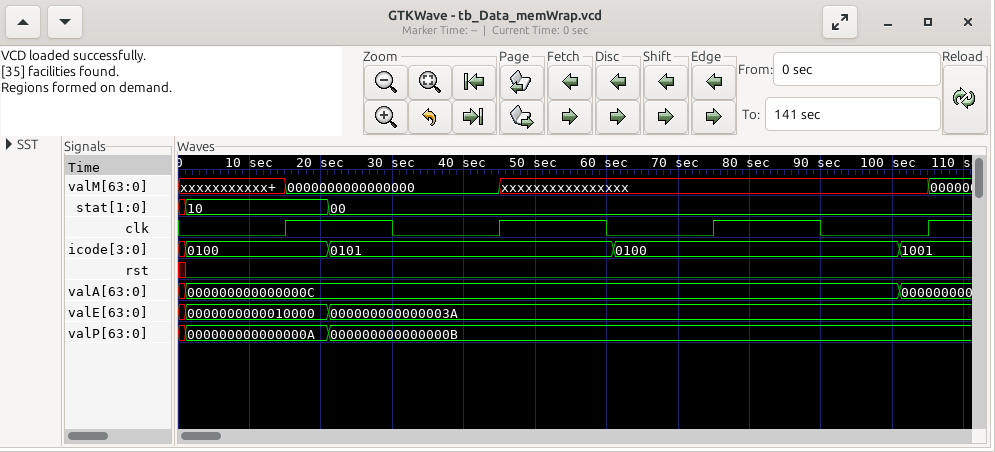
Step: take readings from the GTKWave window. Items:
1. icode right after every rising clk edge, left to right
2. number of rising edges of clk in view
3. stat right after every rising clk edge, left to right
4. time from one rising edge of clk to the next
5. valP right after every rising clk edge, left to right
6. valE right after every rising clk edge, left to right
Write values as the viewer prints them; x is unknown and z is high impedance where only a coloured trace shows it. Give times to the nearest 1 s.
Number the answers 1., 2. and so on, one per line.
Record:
1. 0100, 0101, 0100, 1001
2. 4
3. 10, 00, 00, 00
4. 30 s
5. 000000000000000A, 000000000000000B, 000000000000000B, 000000000000000B
6. 0000000000010000, 000000000000003A, 000000000000003A, 000000000000003A
